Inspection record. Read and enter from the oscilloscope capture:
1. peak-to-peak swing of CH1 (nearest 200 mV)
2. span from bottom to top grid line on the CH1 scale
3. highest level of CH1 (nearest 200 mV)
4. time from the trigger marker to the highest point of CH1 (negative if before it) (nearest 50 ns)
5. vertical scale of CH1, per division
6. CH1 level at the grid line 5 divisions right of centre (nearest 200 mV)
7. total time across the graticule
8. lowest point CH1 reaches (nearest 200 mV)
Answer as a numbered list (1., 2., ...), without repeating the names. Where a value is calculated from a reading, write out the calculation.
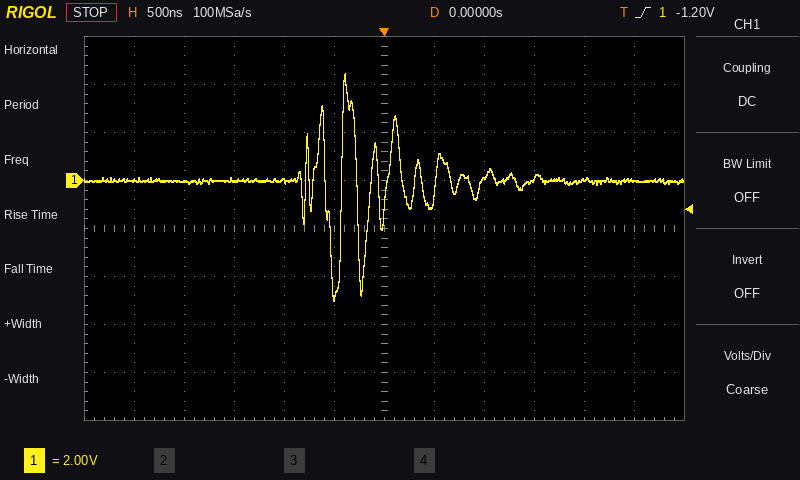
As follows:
1. 4.4 V − (-5.0 V) = 9.4 V
2. 16 V
3. 4.4 V
4. -400 ns
5. 2 V
6. 0.0 V
7. 6 µs
8. -5.0 V
